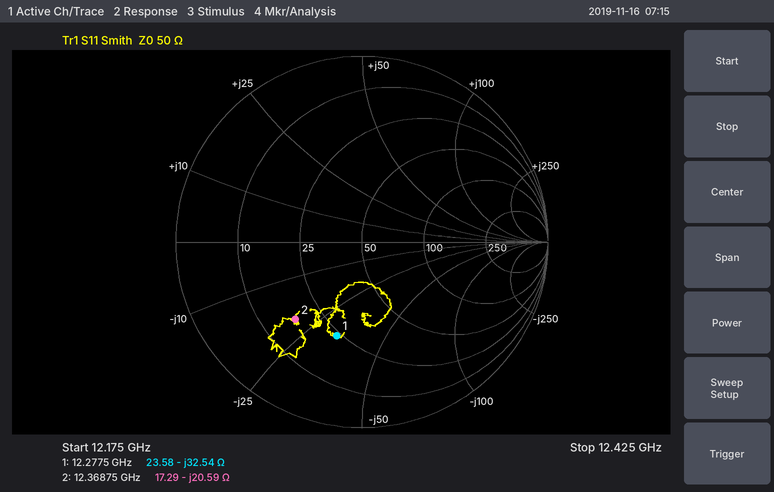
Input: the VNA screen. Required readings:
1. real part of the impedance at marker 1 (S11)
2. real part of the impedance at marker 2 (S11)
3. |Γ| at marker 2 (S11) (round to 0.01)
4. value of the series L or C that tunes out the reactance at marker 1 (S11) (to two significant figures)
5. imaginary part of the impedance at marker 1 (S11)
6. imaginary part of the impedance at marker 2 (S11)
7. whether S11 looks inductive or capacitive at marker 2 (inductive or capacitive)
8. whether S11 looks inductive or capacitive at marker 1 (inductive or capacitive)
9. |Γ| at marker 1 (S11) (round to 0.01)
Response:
23.58 Ω
17.29 Ω
0.55
420 pH
-32.54 Ω
-20.59 Ω
capacitive
capacitive
0.52
